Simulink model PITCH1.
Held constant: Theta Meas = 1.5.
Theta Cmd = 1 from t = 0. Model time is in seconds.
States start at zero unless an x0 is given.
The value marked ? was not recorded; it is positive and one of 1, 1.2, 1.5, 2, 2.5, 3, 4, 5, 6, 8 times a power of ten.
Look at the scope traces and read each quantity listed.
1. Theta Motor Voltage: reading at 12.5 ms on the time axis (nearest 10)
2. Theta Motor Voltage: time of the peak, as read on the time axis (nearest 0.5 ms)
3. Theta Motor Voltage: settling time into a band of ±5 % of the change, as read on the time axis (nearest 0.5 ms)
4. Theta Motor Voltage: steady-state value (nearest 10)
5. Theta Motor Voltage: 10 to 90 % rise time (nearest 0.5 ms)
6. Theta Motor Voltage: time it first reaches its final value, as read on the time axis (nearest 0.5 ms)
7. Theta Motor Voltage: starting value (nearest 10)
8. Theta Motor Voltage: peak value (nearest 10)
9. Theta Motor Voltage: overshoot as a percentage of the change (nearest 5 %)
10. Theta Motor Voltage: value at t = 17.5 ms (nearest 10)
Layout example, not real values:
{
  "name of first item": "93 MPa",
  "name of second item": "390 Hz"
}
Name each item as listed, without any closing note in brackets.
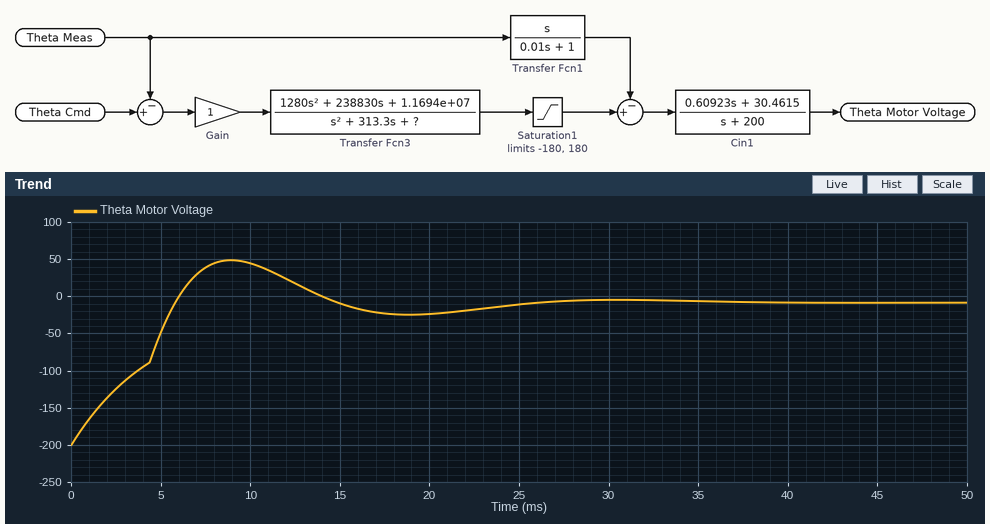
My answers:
{
  "Theta Motor Voltage: reading at 12.5 ms on the time axis": "20",
  "Theta Motor Voltage: time of the peak, as read on the time axis": "9.0 ms",
  "Theta Motor Voltage: settling time into a band of ±5 % of the change, as read on the time axis": "22.5 ms",
  "Theta Motor Voltage: steady-state value": "-10",
  "Theta Motor Voltage: 10 to 90 % rise time": "5.0 ms",
  "Theta Motor Voltage: time it first reaches its final value, as read on the time axis": "6.0 ms",
  "Theta Motor Voltage: starting value": "-200",
  "Theta Motor Voltage: peak value": "50",
  "Theta Motor Voltage: overshoot as a percentage of the change": "30 %",
  "Theta Motor Voltage: value at t = 17.5 ms": "-20"
}
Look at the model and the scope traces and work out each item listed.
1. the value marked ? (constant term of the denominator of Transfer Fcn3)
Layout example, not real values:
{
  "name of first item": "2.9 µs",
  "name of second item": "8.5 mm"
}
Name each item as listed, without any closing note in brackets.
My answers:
{
  "the value marked ?": "100000"
}
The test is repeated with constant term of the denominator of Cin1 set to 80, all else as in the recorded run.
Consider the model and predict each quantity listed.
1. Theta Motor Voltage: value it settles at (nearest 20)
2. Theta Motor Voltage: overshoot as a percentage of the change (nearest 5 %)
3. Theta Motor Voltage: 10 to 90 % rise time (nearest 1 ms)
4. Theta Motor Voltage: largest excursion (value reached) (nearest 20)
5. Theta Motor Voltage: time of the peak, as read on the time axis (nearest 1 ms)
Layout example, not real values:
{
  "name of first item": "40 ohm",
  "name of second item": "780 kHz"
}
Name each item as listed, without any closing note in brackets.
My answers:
{
  "Theta Motor Voltage: value it settles at": "-20",
  "Theta Motor Voltage: overshoot as a percentage of the change": "20 %",
  "Theta Motor Voltage: 10 to 90 % rise time": "5 ms",
  "Theta Motor Voltage: largest excursion (value reached)": "20",
  "Theta Motor Voltage: time of the peak, as read on the time axis": "10 ms"
}
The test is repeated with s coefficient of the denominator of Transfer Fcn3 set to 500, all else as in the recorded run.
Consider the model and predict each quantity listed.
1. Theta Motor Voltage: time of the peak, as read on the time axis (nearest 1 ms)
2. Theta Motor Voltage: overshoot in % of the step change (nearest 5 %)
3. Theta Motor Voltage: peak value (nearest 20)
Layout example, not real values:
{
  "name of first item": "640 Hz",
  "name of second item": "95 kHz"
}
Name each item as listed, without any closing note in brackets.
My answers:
{
  "Theta Motor Voltage: time of the peak, as read on the time axis": "9 ms",
  "Theta Motor Voltage: overshoot in % of the step change": "10 %",
  "Theta Motor Voltage: peak value": "20"
}
